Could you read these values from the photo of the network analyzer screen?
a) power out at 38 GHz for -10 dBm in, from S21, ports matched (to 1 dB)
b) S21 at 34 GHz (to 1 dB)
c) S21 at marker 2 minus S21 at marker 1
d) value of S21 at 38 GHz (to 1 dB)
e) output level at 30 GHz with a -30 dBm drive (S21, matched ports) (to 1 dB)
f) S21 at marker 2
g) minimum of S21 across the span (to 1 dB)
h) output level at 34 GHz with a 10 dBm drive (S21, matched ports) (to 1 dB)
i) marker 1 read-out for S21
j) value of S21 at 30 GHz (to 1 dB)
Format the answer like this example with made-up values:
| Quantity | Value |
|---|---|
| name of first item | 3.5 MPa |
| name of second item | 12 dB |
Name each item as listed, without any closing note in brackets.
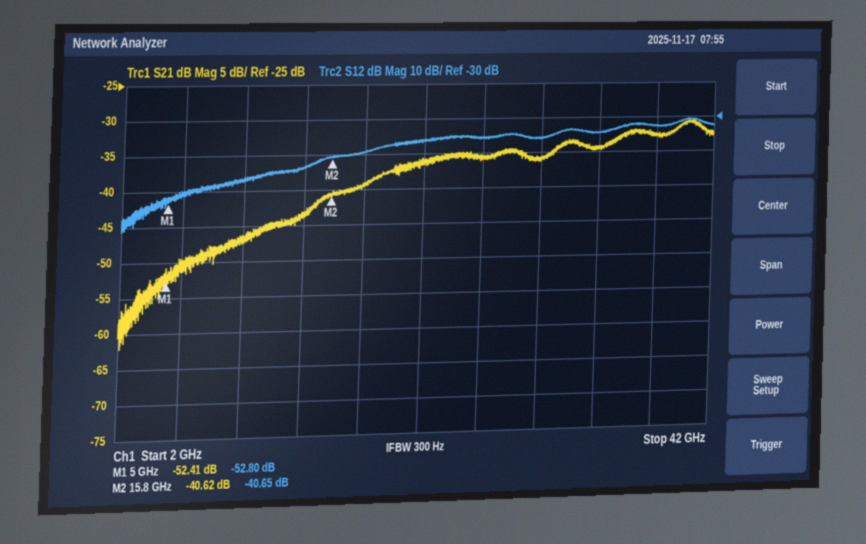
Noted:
| Quantity | Value |
|---|---|
| power out at 38 GHz for -10 dBm in, from S21, ports matched | -43 dBm |
| S21 at 34 GHz | -34 dB |
| S21 at marker 2 minus S21 at marker 1 | 11.79 dB |
| value of S21 at 38 GHz | -33 dB |
| output level at 30 GHz with a -30 dBm drive (S21, matched ports) | -66 dBm |
| S21 at marker 2 | -40.62 dB |
| minimum of S21 across the span | -62 dB |
| output level at 34 GHz with a 10 dBm drive (S21, matched ports) | -24 dBm |
| marker 1 read-out for S21 | -52.41 dB |
| value of S21 at 30 GHz | -36 dB |
